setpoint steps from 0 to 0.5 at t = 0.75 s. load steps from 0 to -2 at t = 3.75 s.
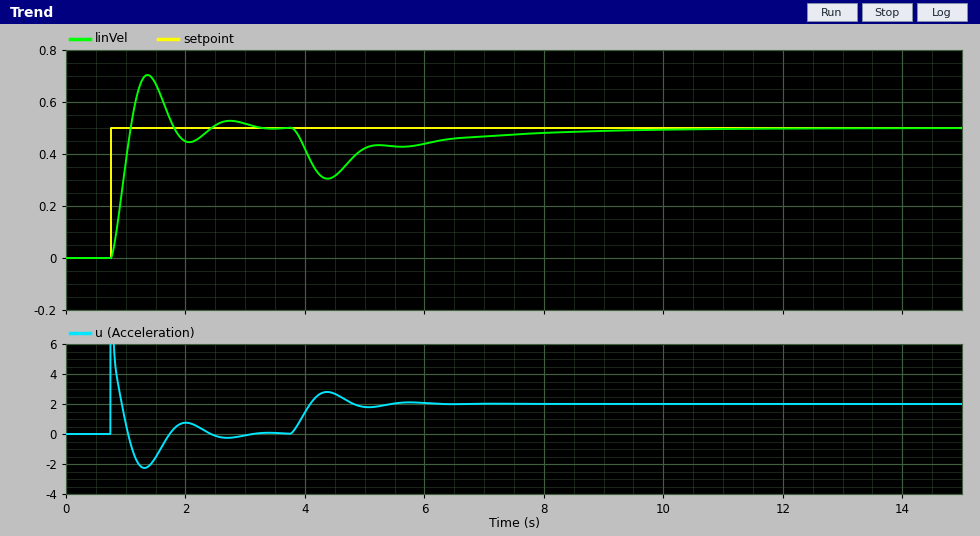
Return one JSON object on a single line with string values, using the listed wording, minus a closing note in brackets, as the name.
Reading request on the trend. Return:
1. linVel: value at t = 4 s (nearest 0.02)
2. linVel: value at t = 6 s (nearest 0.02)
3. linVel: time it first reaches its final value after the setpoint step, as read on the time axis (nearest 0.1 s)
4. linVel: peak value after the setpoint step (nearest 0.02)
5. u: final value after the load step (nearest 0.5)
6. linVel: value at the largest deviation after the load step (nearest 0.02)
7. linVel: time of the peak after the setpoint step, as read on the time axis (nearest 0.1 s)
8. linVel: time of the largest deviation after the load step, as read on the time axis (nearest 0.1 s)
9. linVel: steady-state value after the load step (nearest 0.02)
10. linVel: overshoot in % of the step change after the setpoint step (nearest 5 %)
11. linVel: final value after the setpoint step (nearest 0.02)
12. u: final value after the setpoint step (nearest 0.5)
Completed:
{"linVel: value at t = 4 s": "0.42", "linVel: value at t = 6 s": "0.44", "linVel: time it first reaches its final value after the setpoint step, as read on the time axis": "1.1 s", "linVel: peak value after the setpoint step": "0.70", "u: final value after the load step": "2.0", "linVel: value at the largest deviation after the load step": "0.30", "linVel: time of the peak after the setpoint step, as read on the time axis": "1.4 s", "linVel: time of the largest deviation after the load step, as read on the time axis": "4.4 s", "linVel: steady-state value after the load step": "0.50", "linVel: overshoot in % of the step change after the setpoint step": "40 %", "linVel: final value after the setpoint step": "0.50", "u: final value after the setpoint step": "0.0"}
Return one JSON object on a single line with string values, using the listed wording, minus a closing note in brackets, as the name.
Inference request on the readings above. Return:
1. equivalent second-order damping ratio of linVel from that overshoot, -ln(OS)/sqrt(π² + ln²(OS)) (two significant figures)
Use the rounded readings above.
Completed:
{"equivalent second-order damping ratio of linVel from that overshoot, -ln(OS)/sqrt(π² + ln²(OS))": "0.28"}
